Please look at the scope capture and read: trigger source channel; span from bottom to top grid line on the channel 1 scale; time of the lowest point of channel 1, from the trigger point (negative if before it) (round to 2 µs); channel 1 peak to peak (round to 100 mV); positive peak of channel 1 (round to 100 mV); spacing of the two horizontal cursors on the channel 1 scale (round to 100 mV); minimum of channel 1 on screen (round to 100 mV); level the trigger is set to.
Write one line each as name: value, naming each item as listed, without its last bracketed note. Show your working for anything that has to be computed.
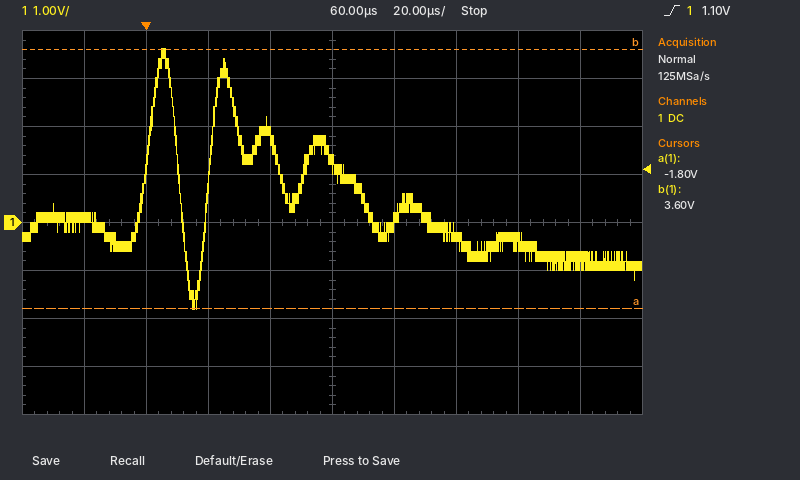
trigger source channel: channel 1
span from bottom to top grid line on the channel 1 scale: 8 V
time of the lowest point of channel 1, from the trigger point (negative if before it): +16 µs
channel 1 peak to peak: 3.6 V − (-1.8 V) = 5.4 V
positive peak of channel 1: 3.6 V
spacing of the two horizontal cursors on the channel 1 scale: 5.4 V
minimum of channel 1 on screen: -1.8 V
level the trigger is set to: 1.10 V
